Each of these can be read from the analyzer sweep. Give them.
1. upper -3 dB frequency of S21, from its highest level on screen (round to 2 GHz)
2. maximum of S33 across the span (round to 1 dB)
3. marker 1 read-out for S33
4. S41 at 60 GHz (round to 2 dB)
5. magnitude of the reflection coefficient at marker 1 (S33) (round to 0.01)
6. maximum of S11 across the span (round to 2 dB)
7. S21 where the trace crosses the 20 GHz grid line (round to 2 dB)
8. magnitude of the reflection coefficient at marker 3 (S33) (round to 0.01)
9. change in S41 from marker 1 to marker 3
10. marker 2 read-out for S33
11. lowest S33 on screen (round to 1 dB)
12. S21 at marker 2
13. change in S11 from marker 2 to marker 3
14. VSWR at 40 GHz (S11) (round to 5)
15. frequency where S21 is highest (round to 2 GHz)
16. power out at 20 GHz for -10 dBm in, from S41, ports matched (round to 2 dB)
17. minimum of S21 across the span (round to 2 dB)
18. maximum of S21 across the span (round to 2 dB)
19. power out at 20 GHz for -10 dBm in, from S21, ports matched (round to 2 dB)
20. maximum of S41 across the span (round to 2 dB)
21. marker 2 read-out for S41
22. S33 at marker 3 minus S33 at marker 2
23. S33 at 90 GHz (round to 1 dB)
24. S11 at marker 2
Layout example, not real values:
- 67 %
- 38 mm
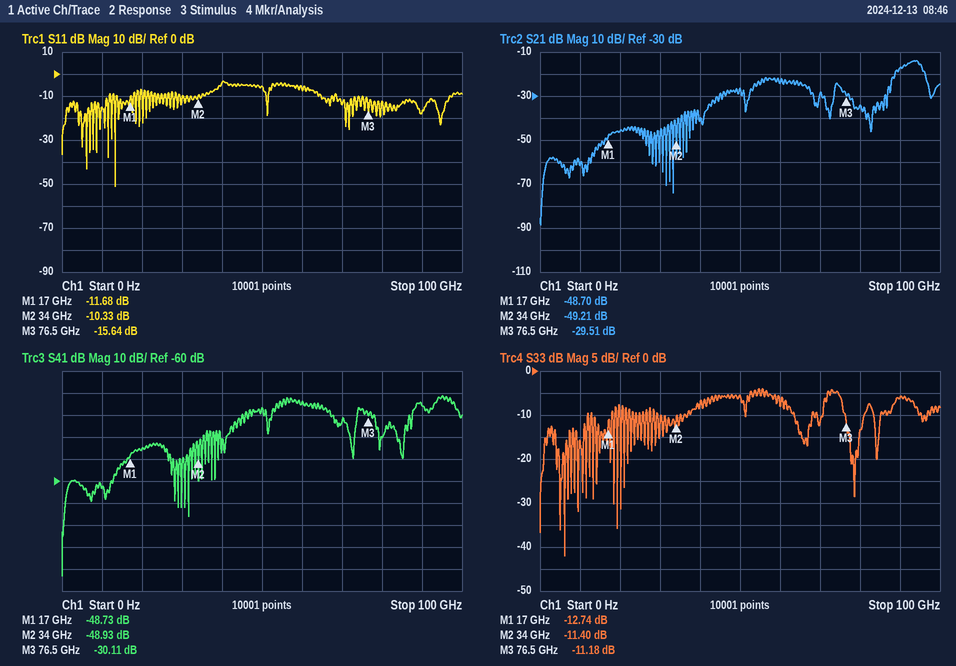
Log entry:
- 96 GHz
- -4 dB
- -12.74 dB
- -24 dB
- 0.23
- -4 dB
- -46 dB
- 0.28
- 18.62 dB
- -11.40 dB
- -42 dB
- -49.21 dB
- -5.31 dB
- 5
- 94 GHz
- -56 dBm
- -88 dB
- -14 dB
- -56 dBm
- -22 dB
- -48.93 dB
- 0.22 dB
- -6 dB
- -10.33 dB
